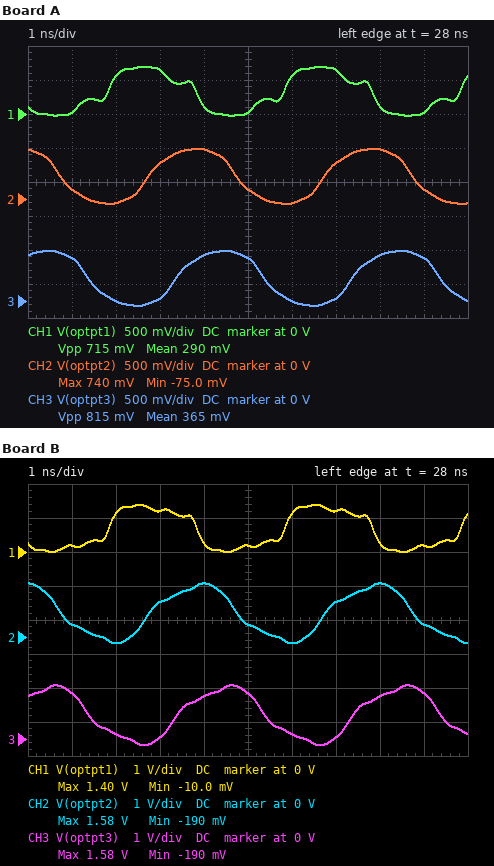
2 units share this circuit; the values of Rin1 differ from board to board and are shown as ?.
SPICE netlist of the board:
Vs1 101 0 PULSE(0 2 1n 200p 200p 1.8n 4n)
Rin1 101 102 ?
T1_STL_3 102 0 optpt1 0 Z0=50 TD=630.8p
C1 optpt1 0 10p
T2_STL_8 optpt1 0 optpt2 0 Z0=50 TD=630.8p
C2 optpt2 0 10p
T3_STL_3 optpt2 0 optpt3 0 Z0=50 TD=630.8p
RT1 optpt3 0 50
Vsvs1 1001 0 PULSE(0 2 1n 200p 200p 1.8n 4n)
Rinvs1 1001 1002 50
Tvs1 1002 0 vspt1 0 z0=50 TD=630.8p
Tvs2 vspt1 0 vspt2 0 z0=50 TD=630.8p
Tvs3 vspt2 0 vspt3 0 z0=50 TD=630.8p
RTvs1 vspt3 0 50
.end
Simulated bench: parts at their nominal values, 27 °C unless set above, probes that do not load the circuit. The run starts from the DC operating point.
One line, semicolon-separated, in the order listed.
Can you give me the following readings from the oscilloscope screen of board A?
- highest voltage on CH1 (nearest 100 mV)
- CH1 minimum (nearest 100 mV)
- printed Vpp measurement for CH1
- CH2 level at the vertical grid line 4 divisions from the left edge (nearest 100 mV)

700 mV; 0 V; 715 mV; 700 mV
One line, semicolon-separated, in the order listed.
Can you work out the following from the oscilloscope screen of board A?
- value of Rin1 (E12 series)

100 Ω
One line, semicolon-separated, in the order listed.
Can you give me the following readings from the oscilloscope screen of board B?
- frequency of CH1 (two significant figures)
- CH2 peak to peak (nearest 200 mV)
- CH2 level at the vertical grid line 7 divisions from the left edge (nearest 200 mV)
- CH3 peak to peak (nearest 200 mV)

250 MHz; 1.8 V; 1.0 V; 1.8 V
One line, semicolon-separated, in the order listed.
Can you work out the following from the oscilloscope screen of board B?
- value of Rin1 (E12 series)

22 Ω
